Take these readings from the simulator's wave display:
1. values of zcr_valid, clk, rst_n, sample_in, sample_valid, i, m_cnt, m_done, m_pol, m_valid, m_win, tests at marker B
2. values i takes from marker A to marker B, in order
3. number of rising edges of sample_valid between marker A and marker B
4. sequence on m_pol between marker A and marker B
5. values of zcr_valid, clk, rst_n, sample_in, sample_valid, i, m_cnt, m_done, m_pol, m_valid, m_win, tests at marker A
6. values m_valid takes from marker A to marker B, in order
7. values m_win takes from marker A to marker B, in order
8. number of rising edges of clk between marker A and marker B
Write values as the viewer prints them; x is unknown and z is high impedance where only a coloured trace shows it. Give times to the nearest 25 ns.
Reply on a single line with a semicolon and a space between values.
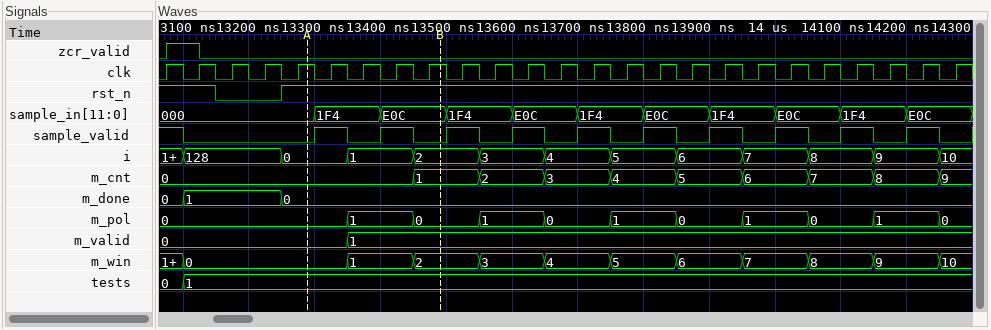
zcr_valid=0, clk=1, rst_n=1, sample_in=E0C, sample_valid=0, i=2, m_cnt=1, m_done=0, m_pol=0, m_valid=1, m_win=2, tests=1; 0, 1, 2; 2; 0, 1, 0; zcr_valid=0, clk=1, rst_n=1, sample_in=000, sample_valid=0, i=0, m_cnt=0, m_done=0, m_pol=0, m_valid=0, m_win=0, tests=1; 0, 1; 0, 1, 2; 4
